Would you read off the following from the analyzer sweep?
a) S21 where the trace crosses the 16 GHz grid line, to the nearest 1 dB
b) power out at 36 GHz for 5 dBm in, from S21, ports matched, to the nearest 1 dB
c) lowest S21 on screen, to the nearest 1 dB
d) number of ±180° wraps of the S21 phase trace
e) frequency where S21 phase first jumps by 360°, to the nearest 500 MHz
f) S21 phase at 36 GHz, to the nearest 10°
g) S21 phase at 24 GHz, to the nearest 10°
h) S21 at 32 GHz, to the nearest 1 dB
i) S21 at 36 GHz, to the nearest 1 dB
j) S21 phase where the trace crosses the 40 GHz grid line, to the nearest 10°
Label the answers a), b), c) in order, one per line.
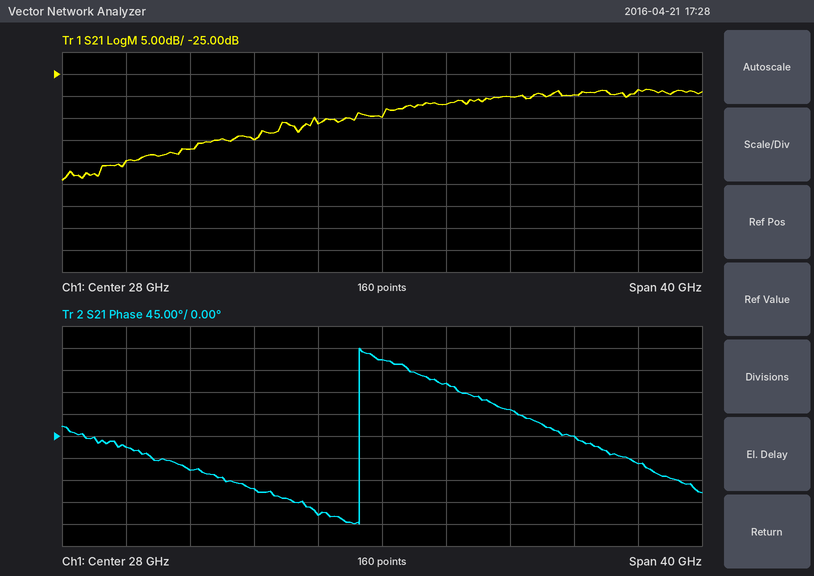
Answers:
a) -42 dB
b) -25 dBm
c) -49 dB
d) 1
e) 26.5 GHz
f) 50°
g) -160°
h) -32 dB
i) -30 dB
j) 0°
